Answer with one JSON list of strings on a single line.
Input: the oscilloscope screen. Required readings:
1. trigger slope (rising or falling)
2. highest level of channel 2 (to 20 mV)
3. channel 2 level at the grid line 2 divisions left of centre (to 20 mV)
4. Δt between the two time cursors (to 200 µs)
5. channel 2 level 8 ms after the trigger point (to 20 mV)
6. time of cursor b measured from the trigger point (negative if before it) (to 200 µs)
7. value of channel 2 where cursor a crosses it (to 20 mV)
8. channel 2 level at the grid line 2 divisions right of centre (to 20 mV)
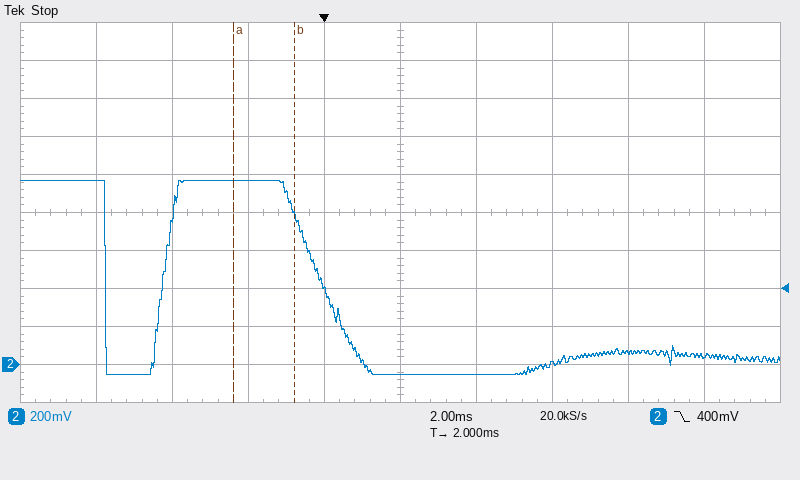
["falling", "960 mV", "960 mV", "1.6 ms", "60 mV", "-800 µs", "960 mV", "0 mV"]
